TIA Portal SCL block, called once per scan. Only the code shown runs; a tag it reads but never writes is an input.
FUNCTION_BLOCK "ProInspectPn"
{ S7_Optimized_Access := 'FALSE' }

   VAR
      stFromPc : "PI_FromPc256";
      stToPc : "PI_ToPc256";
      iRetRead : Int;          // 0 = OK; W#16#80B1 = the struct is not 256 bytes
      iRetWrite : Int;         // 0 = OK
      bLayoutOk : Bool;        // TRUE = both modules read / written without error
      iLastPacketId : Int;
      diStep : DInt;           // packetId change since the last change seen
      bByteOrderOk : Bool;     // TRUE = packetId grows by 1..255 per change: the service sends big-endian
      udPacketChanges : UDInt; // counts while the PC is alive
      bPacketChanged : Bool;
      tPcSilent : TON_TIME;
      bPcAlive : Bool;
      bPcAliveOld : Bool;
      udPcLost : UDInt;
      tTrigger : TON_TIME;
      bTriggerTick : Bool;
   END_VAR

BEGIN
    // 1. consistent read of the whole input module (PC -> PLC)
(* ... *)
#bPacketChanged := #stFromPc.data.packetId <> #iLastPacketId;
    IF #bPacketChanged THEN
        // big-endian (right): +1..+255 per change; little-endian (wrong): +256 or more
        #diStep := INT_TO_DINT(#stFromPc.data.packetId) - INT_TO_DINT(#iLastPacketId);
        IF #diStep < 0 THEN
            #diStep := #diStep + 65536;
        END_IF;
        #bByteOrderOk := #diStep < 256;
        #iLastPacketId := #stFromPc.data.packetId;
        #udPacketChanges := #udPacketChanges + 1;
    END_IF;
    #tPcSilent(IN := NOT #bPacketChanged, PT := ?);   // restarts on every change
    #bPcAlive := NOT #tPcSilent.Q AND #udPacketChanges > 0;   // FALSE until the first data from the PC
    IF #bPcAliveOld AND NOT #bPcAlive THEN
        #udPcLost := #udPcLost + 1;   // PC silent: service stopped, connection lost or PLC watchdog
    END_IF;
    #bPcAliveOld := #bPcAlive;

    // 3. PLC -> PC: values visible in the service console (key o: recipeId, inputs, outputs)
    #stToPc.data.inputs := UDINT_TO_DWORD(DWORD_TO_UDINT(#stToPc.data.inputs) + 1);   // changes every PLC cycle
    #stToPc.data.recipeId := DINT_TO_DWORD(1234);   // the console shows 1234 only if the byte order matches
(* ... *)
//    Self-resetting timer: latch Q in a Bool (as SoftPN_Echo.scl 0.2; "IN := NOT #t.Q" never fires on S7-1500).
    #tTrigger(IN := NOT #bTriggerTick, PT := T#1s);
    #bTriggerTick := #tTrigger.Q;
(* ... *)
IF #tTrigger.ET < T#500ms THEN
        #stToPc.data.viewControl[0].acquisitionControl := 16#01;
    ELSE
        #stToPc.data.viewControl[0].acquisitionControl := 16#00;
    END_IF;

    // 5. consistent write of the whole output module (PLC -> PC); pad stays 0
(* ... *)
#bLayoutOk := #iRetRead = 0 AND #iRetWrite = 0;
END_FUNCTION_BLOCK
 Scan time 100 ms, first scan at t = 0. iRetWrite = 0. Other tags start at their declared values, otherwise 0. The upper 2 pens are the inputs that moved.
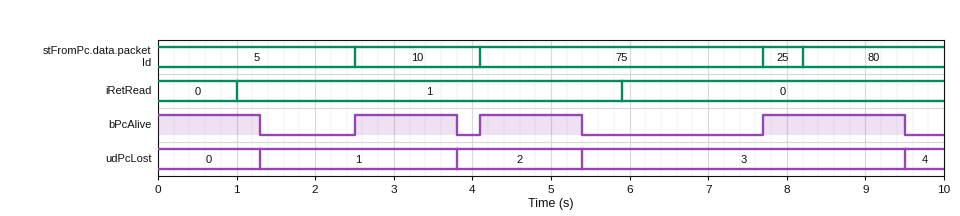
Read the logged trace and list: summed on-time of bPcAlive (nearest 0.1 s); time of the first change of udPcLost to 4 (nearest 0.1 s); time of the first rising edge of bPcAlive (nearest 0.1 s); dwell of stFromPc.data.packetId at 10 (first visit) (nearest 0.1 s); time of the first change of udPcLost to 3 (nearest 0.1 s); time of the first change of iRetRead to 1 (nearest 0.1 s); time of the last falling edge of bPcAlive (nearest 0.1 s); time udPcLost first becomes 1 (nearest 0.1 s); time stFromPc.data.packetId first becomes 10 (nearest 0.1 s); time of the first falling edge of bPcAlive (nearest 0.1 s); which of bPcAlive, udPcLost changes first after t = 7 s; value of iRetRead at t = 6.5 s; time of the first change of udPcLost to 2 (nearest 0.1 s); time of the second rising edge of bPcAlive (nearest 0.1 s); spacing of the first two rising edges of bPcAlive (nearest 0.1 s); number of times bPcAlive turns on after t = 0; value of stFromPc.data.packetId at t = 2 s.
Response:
5.7 s
9.5 s
2.5 s
1.6 s
5.4 s
1.0 s
9.5 s
1.3 s
2.5 s
1.3 s
bPcAlive
0
3.8 s
4.1 s
1.6 s
3
5
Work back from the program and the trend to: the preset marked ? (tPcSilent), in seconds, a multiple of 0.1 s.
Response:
1.2 s
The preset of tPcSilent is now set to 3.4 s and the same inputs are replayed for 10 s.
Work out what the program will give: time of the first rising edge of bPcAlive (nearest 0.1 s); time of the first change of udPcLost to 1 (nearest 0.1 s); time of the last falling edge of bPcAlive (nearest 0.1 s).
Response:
7.7 s
7.6 s
7.6 s
